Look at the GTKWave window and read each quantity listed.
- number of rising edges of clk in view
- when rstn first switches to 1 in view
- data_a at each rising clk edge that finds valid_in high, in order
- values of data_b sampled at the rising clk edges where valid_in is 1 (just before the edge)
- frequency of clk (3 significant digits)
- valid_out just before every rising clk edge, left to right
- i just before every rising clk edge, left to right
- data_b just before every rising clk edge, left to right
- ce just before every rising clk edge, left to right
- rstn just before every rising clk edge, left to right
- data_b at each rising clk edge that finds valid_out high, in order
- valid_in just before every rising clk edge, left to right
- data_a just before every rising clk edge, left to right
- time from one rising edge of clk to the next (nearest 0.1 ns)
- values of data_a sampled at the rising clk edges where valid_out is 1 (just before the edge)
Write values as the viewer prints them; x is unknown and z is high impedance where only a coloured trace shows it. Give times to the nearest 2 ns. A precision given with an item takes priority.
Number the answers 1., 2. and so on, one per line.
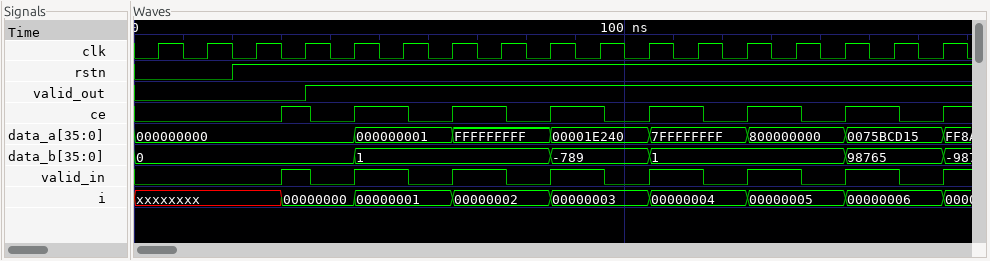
1. 17
2. 20 ns
3. 000000000, 000000001, FFFFFFFFF, 00001E240, 7FFFFFFFF, 800000000, 0075BCD15
4. 0, 1, 1, -789, 1, 1, 98765
5. 100 MHz
6. 0 0 0 0 1 1 1 1 1 1 1 1 1 1 1 1 1
7. xxxxxxxx, xxxxxxxx, xxxxxxxx, 00000000, 00000000, 00000001, 00000001, 00000002, 00000002, 00000003, 00000003, 00000004, 00000004, 00000005, 00000005, 00000006, 00000006
8. 0, 0, 0, 0, 0, 1, 1, 1, 1, -789, -789, 1, 1, 1, 1, 98765, 98765
9. 0 0 0 1 0 1 0 1 0 1 0 1 0 1 0 1 0
10. 0 0 1 1 1 1 1 1 1 1 1 1 1 1 1 1 1
11. 0, 1, 1, 1, 1, -789, -789, 1, 1, 1, 1, 98765, 98765
12. 0 0 0 1 0 1 0 1 0 1 0 1 0 1 0 1 0
13. 000000000, 000000000, 000000000, 000000000, 000000000, 000000001, 000000001, FFFFFFFFF, FFFFFFFFF, 00001E240, 00001E240, 7FFFFFFFF, 7FFFFFFFF, 800000000, 800000000, 0075BCD15, 0075BCD15
14. 10 ns
15. 000000000, 000000001, 000000001, FFFFFFFFF, FFFFFFFFF, 00001E240, 00001E240, 7FFFFFFFF, 7FFFFFFFF, 800000000, 800000000, 0075BCD15, 0075BCD15
